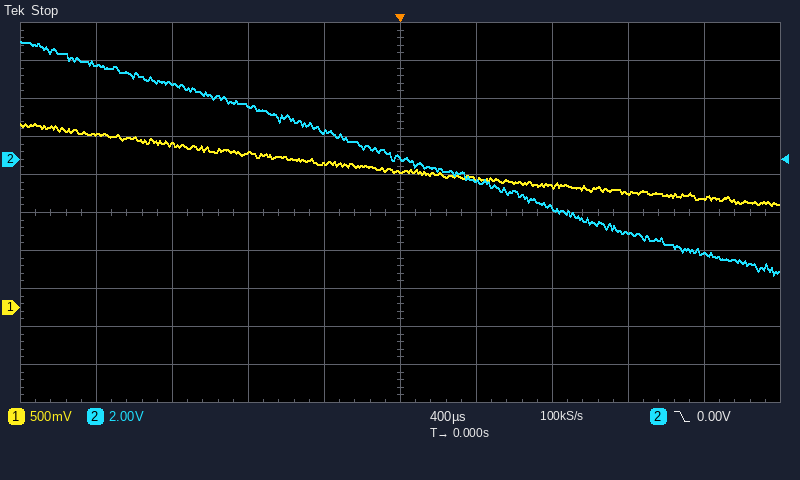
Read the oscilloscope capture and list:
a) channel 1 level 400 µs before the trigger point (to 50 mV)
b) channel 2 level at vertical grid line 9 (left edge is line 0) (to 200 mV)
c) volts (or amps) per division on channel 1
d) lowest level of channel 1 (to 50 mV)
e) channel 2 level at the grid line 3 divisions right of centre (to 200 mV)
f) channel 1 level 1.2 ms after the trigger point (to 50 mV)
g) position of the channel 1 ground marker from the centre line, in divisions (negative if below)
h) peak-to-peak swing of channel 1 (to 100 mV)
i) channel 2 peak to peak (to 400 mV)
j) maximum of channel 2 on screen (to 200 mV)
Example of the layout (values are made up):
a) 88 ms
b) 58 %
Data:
a) 1.90 V
b) -5.0 V
c) 500 mV
d) 1.35 V
e) -3.8 V
f) 1.50 V
g) -2.5 div
h) 1.10 V
i) 12.4 V
j) 6.2 V
